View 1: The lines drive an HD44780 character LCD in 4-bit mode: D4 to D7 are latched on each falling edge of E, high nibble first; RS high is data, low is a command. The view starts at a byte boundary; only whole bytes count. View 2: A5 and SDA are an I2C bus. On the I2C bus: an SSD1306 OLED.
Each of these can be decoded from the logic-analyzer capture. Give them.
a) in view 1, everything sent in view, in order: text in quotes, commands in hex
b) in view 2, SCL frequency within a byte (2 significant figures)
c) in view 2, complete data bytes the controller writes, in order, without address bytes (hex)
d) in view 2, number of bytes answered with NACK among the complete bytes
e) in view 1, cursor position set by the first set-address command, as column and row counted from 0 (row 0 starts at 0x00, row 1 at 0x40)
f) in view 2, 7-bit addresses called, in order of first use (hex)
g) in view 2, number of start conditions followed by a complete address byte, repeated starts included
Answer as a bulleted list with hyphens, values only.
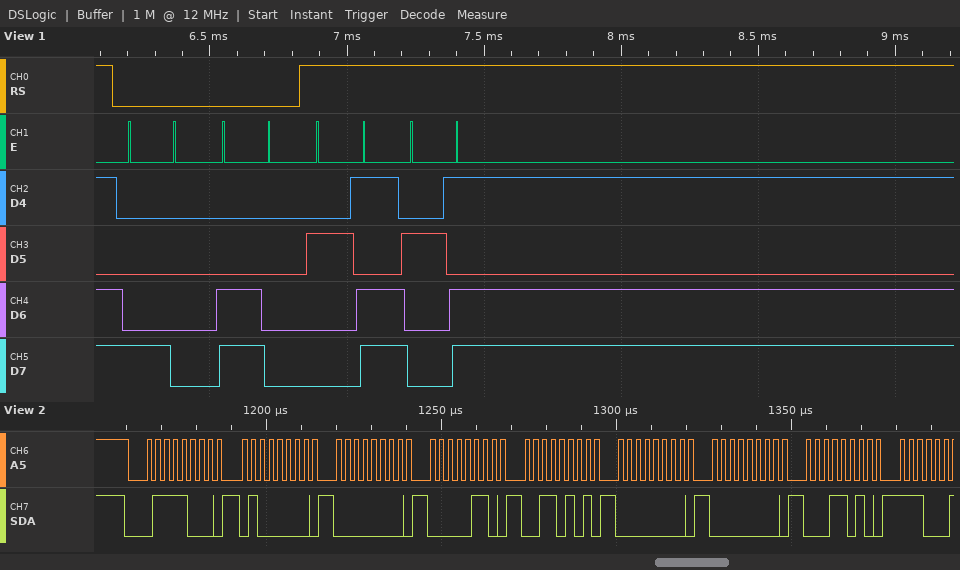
- 0x80 0xC0 "--"
- 400 kHz
- 40 00 06 35 00 00 1A
- 0
- column 0, row 0
- 0x3C
- 1
